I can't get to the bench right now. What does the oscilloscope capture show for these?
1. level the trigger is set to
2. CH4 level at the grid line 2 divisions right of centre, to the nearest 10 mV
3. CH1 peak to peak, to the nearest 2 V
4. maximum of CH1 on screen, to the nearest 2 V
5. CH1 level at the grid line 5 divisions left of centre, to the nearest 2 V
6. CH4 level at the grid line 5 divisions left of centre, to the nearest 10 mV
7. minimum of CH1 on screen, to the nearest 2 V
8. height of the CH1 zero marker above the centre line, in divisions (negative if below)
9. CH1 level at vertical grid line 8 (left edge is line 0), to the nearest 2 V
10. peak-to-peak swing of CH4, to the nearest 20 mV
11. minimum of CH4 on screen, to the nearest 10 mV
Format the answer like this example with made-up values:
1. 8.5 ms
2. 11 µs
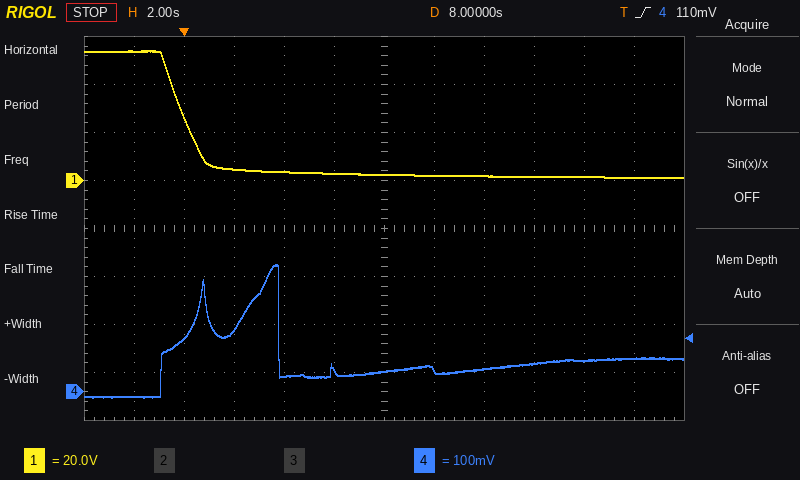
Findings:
1. 110 mV
2. 50 mV
3. 52 V
4. 54 V
5. 54 V
6. -10 mV
7. 2 V
8. +1.0 div
9. 2 V
10. 280 mV
11. -10 mV
